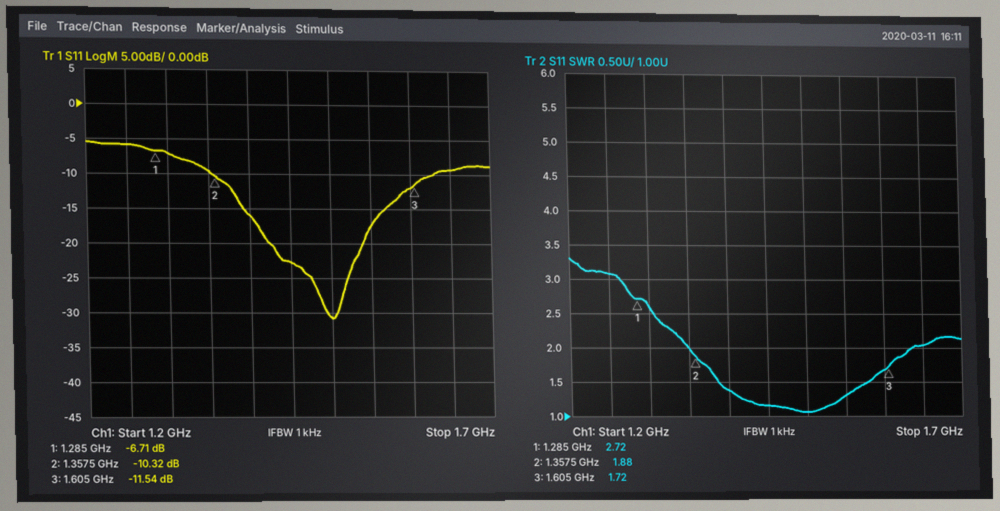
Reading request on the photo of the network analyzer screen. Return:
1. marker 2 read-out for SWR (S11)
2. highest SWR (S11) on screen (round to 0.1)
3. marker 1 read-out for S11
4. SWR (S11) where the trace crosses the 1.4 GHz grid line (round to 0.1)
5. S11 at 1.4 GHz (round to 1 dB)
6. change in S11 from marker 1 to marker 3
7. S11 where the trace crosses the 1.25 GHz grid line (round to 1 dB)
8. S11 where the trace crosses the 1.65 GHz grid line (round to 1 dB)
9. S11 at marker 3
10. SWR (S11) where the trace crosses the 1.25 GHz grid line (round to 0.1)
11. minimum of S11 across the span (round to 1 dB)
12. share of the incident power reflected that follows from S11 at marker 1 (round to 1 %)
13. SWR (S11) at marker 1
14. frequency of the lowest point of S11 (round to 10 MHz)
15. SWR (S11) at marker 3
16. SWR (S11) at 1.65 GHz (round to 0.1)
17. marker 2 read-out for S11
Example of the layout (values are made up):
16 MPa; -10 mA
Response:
1.88; 3.3; -6.71 dB; 1.4; -16 dB; -4.83 dB; -6 dB; -9 dB; -11.54 dB; 3.1; -31 dB; 21 %; 2.72; 1.50 GHz; 1.72; 2.0; -10.32 dB
